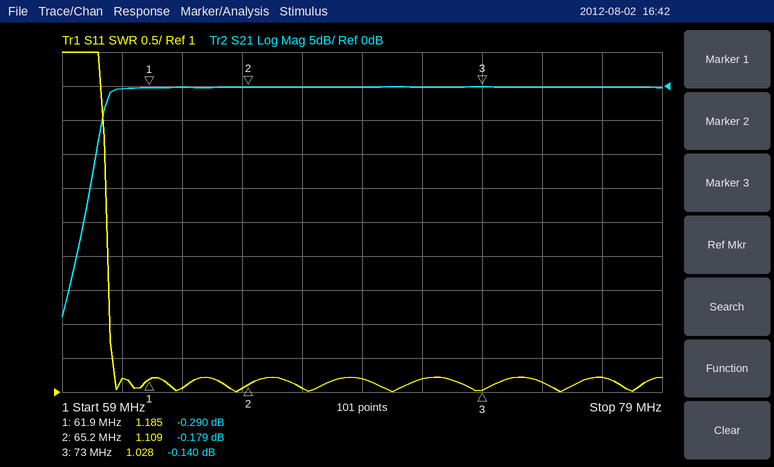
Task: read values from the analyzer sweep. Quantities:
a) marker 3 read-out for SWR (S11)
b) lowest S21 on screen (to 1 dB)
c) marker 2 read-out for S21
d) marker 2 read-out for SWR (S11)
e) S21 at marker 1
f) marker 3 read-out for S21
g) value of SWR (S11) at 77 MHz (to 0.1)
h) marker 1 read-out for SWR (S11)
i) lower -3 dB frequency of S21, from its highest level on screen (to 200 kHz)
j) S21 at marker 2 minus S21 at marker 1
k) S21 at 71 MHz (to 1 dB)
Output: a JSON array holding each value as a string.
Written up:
["1.028", "-34 dB", "-0.179 dB", "1.109", "-0.290 dB", "-0.140 dB", "1.2", "1.185", "60.4 MHz", "0.111 dB", "0 dB"]
